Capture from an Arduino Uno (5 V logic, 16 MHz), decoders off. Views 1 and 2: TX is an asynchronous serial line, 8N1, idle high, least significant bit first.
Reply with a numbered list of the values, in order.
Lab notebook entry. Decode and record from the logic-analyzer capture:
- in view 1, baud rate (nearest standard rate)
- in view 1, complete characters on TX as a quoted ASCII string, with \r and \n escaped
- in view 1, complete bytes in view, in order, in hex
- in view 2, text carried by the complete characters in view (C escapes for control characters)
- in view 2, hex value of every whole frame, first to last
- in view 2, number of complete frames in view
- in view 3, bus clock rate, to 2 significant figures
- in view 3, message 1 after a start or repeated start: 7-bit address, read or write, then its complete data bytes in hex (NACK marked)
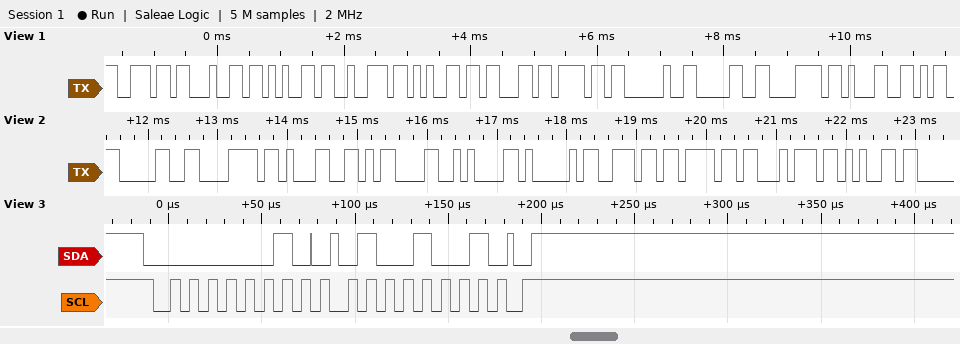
1. 9600 baud
2. "ndereco 0x1"
3. 6E 64 65 72 65 63 6F 20 30 78 31
4. "0x1\r\nAnote"
5. 30 78 31 0D 0A 41 6E 6F 74 65
6. 10
7. 100 kHz
8. 0x01 write: 49
